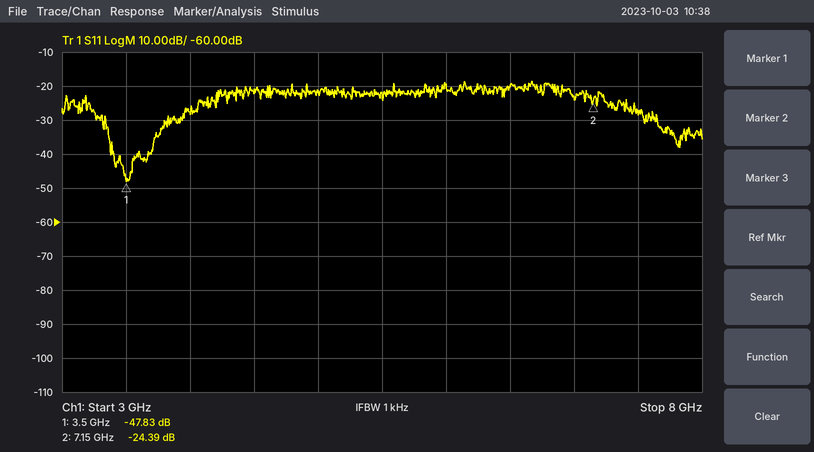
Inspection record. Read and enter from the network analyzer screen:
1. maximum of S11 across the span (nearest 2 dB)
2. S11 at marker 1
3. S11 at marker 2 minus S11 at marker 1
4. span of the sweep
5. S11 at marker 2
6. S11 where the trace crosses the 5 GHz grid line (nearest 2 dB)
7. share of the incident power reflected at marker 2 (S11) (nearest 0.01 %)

-18 dB
-47.83 dB
23.44 dB
5 GHz
-24.39 dB
-22 dB
0.36 %
